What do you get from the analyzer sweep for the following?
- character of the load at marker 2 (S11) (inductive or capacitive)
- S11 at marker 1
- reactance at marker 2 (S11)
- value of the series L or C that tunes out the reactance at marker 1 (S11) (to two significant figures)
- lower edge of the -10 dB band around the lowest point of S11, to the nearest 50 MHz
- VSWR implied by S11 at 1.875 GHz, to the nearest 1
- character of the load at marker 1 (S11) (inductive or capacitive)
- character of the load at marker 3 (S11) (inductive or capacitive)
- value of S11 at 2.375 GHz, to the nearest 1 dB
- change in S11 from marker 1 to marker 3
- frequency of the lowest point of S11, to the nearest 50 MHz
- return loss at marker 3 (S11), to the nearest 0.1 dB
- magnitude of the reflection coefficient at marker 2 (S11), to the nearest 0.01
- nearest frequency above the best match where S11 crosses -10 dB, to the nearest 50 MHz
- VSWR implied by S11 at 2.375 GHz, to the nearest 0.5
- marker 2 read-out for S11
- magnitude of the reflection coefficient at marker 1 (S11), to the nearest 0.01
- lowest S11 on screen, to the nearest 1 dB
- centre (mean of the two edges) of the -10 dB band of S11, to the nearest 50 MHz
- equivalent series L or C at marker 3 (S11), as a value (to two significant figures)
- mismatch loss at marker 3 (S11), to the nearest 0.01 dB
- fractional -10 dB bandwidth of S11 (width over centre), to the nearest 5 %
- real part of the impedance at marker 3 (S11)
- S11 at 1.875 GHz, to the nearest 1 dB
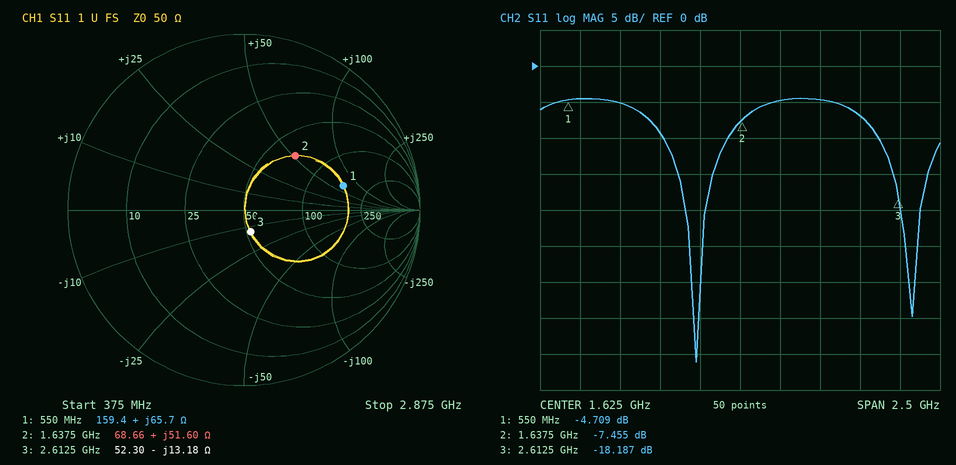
inductive
-4.709 dB
+51.60 Ω
4.4 pF
1.15 GHz
4
inductive
capacitive
-7 dB
-13.478 dB
1.35 GHz
17.7 dB
0.42
1.55 GHz
2.5
-7.455 dB
0.58
-41 dB
1.35 GHz
4.6 pF
0.07 dB
30 %
52.30 Ω
-5 dB
